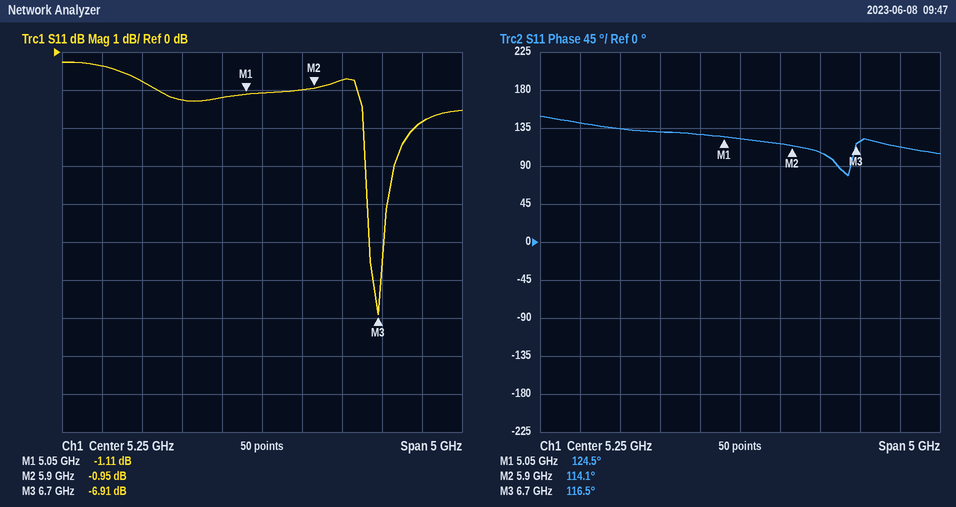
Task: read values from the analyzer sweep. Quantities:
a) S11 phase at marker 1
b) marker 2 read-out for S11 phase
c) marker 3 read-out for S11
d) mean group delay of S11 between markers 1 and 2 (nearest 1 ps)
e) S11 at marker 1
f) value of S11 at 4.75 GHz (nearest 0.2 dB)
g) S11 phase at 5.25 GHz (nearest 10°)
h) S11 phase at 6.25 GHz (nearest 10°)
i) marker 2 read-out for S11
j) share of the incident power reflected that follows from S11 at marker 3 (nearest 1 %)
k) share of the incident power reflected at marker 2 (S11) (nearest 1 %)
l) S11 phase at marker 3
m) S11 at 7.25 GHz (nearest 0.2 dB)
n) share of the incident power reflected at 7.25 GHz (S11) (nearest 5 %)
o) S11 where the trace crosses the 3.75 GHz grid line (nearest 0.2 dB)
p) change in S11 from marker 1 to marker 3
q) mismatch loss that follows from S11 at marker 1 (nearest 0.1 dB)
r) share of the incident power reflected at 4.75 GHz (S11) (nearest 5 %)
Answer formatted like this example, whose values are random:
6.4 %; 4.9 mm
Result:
124.5°; 114.1°; -6.91 dB; 34 ps; -1.11 dB; -1.2 dB; 120°; 110°; -0.95 dB; 20 %; 80 %; 116.5°; -1.8 dB; 65 %; -0.8 dB; -5.80 dB; 6.5 dB; 75 %
